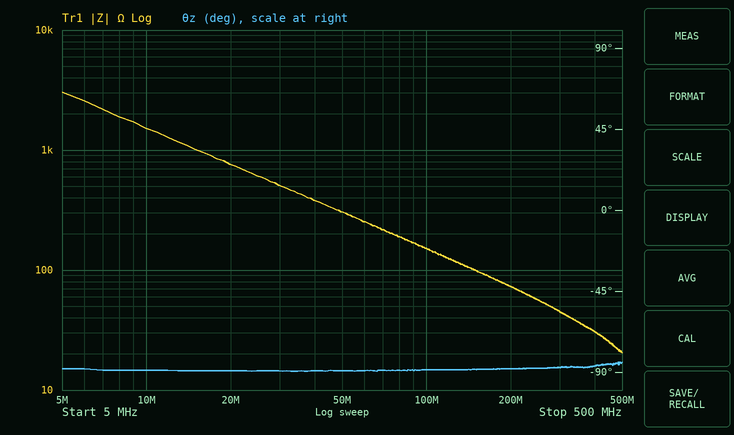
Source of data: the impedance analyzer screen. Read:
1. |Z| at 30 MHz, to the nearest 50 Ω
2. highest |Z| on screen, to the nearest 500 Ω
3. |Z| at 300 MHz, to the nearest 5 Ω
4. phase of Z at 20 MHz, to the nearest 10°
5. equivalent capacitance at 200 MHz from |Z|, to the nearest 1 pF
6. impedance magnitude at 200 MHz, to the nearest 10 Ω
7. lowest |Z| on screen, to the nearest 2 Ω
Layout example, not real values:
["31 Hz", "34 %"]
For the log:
["500 Ω", "3.0 kΩ", "45 Ω", "-90°", "11 pF", "70 Ω", "20 Ω"]
